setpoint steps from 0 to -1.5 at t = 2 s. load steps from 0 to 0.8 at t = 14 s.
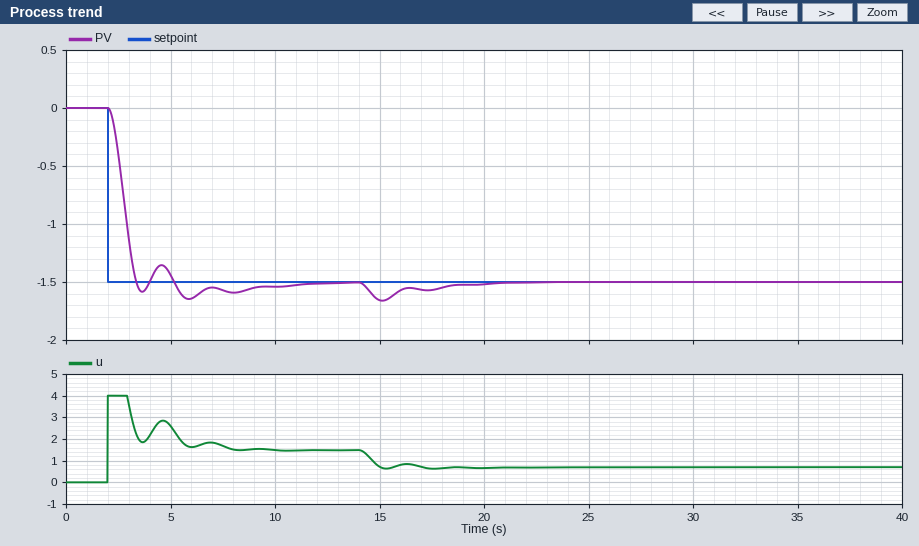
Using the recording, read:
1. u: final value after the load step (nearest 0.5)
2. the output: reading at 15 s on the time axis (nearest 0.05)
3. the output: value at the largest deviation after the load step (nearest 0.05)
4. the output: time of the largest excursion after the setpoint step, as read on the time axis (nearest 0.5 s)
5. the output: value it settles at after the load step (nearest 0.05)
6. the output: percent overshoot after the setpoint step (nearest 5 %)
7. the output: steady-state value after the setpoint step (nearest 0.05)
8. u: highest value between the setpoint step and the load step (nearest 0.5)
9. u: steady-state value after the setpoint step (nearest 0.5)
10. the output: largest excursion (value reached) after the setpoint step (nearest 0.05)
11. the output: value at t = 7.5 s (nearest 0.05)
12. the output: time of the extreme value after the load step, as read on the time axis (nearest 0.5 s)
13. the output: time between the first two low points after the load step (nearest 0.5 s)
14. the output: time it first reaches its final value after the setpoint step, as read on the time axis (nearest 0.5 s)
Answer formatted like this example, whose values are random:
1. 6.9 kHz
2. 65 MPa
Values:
1. 0.5
2. -1.65
3. -1.65
4. 6.0 s
5. -1.50
6. 10 %
7. -1.50
8. 4.0
9. 1.5
10. -1.65
11. -1.55
12. 15.0 s
13. 2.0 s
14. 3.5 s
